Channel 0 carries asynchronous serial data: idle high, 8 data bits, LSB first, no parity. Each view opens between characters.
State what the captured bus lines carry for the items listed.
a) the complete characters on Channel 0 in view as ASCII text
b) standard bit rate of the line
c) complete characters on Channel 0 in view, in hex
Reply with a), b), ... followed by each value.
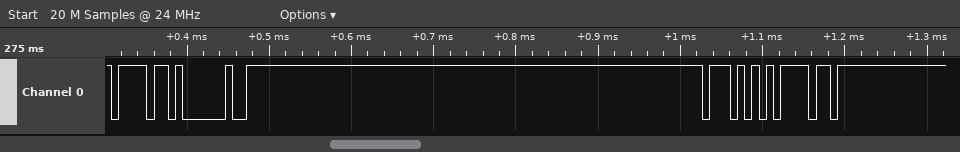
a) "o Wo"
b) 115200 baud
c) 6F, 20, 57, 6F
